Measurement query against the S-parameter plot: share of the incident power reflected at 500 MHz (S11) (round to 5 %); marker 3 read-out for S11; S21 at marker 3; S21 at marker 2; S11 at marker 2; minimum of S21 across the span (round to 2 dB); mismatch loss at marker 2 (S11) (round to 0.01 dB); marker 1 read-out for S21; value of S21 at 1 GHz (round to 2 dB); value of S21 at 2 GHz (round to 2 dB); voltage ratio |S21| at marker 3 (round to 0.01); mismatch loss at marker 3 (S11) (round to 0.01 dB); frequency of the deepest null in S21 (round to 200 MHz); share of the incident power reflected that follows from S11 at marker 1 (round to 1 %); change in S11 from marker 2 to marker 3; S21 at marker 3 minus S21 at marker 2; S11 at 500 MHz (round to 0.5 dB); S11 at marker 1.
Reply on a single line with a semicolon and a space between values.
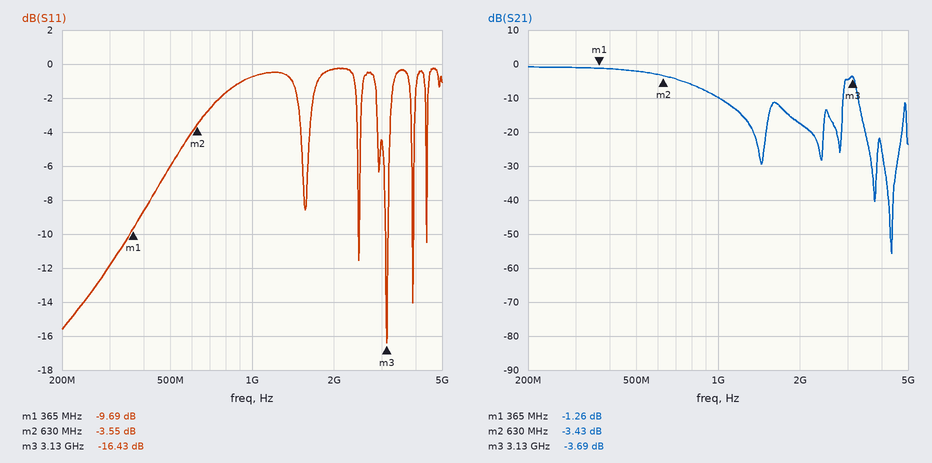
25 %; -16.43 dB; -3.69 dB; -3.43 dB; -3.55 dB; -56 dB; 2.53 dB; -1.26 dB; -10 dB; -18 dB; 0.65; 0.10 dB; 4.4 GHz; 11 %; -12.88 dB; -0.26 dB; -6.0 dB; -9.69 dB
